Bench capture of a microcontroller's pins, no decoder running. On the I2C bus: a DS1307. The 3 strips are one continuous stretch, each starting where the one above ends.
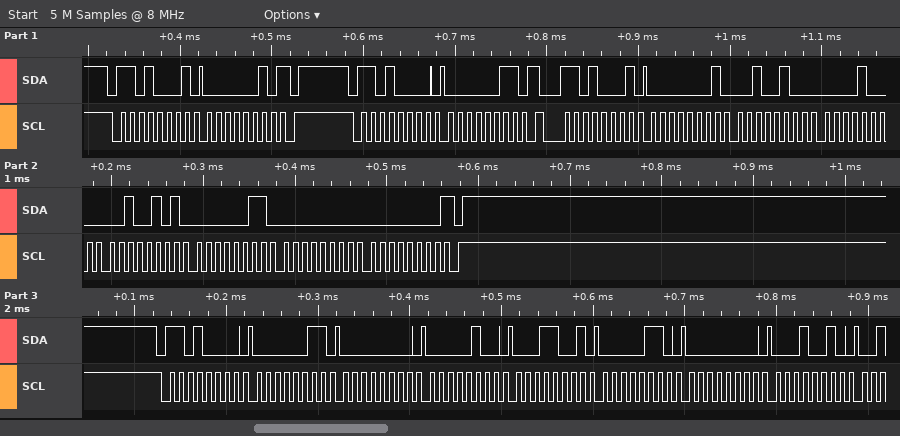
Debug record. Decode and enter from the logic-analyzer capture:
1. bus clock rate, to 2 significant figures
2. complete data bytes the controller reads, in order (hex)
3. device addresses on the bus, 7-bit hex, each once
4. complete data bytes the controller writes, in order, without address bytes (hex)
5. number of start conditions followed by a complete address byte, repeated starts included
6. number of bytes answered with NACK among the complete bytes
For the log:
100 kHz
02 01 24 08 25 03 00 00
0x68
03 03 00 04 19 06 00 12
4
2
